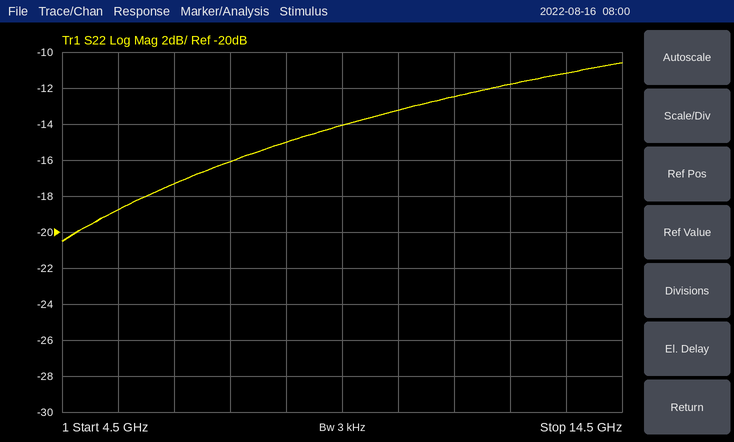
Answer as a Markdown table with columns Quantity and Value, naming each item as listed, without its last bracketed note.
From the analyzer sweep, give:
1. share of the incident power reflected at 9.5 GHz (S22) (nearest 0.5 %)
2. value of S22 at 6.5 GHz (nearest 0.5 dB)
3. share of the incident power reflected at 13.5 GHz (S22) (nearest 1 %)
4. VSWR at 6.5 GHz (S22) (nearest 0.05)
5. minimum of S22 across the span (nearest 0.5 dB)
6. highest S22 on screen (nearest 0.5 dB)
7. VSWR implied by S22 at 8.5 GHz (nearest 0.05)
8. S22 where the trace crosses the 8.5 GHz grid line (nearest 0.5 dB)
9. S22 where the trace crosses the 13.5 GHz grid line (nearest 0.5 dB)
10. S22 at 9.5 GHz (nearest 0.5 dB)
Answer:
| Quantity | Value |
|---|---|
| share of the incident power reflected at 9.5 GHz (S22) | 4.0 % |
| value of S22 at 6.5 GHz | -17.5 dB |
| share of the incident power reflected at 13.5 GHz (S22) | 8 % |
| VSWR at 6.5 GHz (S22) | 1.30 |
| minimum of S22 across the span | -20.5 dB |
| highest S22 on screen | -10.5 dB |
| VSWR implied by S22 at 8.5 GHz | 1.45 |
| S22 where the trace crosses the 8.5 GHz grid line | -15.0 dB |
| S22 where the trace crosses the 13.5 GHz grid line | -11.0 dB |
| S22 at 9.5 GHz | -14.0 dB |
